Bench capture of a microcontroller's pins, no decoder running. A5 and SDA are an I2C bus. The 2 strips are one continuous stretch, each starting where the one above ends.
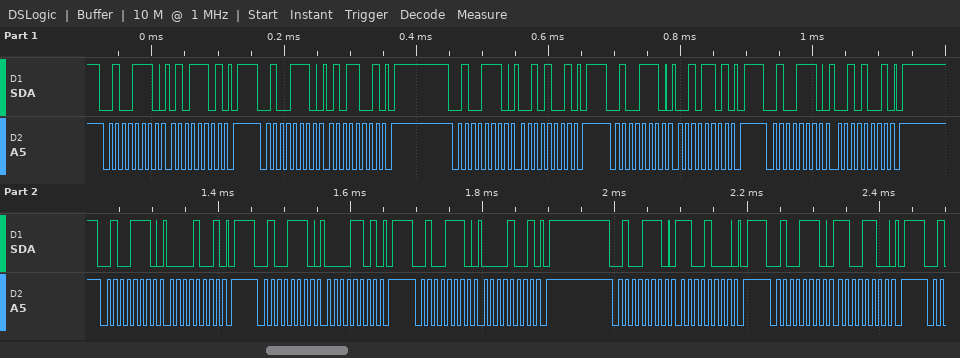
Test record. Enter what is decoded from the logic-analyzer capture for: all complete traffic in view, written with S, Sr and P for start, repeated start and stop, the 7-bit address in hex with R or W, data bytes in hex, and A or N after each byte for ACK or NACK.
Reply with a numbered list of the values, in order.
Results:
1. S 27W A 5D A P S 27W A 59 A P S 27W A 29 A P S 27W A 2D A P S 27W A 29 A P S 27W A 09 A P S 27W A 0D A P S 27W A 09 A P S 27W A C8 A P S 27W A CC A P
